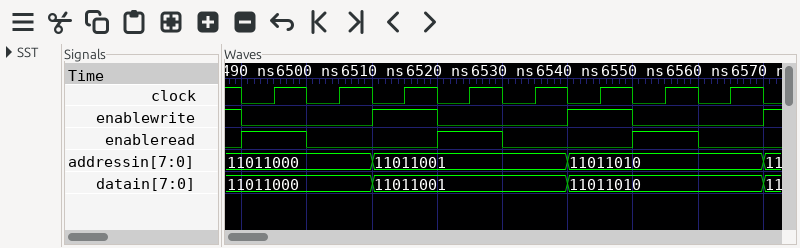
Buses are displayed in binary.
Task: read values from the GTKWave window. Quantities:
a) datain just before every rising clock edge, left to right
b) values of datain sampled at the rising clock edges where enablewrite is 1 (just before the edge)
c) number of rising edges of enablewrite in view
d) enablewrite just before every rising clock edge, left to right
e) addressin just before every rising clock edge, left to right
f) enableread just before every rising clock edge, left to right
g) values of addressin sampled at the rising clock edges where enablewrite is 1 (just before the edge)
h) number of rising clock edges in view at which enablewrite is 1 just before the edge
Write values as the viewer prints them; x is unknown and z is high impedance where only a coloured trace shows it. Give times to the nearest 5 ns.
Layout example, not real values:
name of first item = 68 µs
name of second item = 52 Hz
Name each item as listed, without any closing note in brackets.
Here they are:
datain just before every rising clock edge, left to right = 11011000, 11011000, 11011001, 11011001, 11011001, 11011010, 11011010, 11011010
values of datain sampled at the rising clock edges where enablewrite is 1 = 11011001, 11011010
number of rising edges of enablewrite in view = 3
enablewrite just before every rising clock edge, left to right = 0 0 1 0 0 1 0 0
addressin just before every rising clock edge, left to right = 11011000, 11011000, 11011001, 11011001, 11011001, 11011010, 11011010, 11011010
enableread just before every rising clock edge, left to right = 1 0 0 1 0 0 1 0
values of addressin sampled at the rising clock edges where enablewrite is 1 = 11011001, 11011010
number of rising clock edges in view at which enablewrite is 1 just before the edge = 2
